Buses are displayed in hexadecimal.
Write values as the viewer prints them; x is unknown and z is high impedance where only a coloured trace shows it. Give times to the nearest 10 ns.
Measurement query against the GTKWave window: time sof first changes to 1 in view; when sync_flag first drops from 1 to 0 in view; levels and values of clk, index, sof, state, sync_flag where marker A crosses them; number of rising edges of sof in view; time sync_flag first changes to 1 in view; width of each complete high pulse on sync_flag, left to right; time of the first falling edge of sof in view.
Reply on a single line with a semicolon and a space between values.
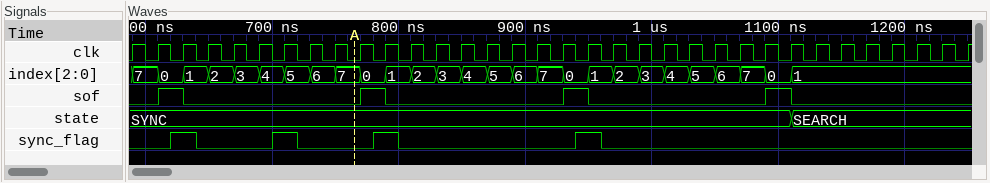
610 ns; 640 ns; clk=0, index=7, sof=0, state=SYNC, sync_flag=0; 4; 620 ns; 20 ns, 20 ns, 20 ns, 20 ns; 630 ns
